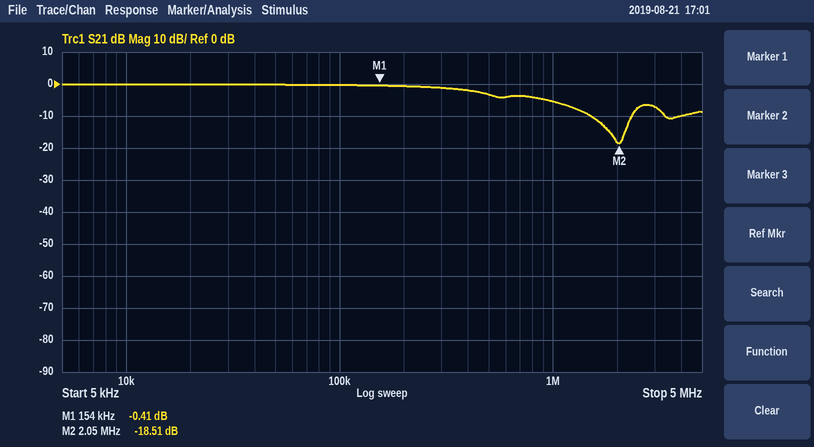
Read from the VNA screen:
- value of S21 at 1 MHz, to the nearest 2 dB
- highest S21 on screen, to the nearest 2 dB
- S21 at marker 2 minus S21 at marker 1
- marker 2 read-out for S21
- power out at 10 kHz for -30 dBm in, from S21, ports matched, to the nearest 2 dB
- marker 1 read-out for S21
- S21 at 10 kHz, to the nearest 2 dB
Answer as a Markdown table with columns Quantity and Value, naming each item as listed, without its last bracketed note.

| Quantity | Value |
|---|---|
| value of S21 at 1 MHz, to the nearest 2 dB | -6 dB |
| highest S21 on screen, to the nearest 2 dB | 0 dB |
| S21 at marker 2 minus S21 at marker 1 | -18.10 dB |
| marker 2 read-out for S21 | -18.51 dB |
| power out at 10 kHz for -30 dBm in, from S21, ports matched, to the nearest 2 dB | -30 dBm |
| marker 1 read-out for S21 | -0.41 dB |
| S21 at 10 kHz, to the nearest 2 dB | 0 dB |
